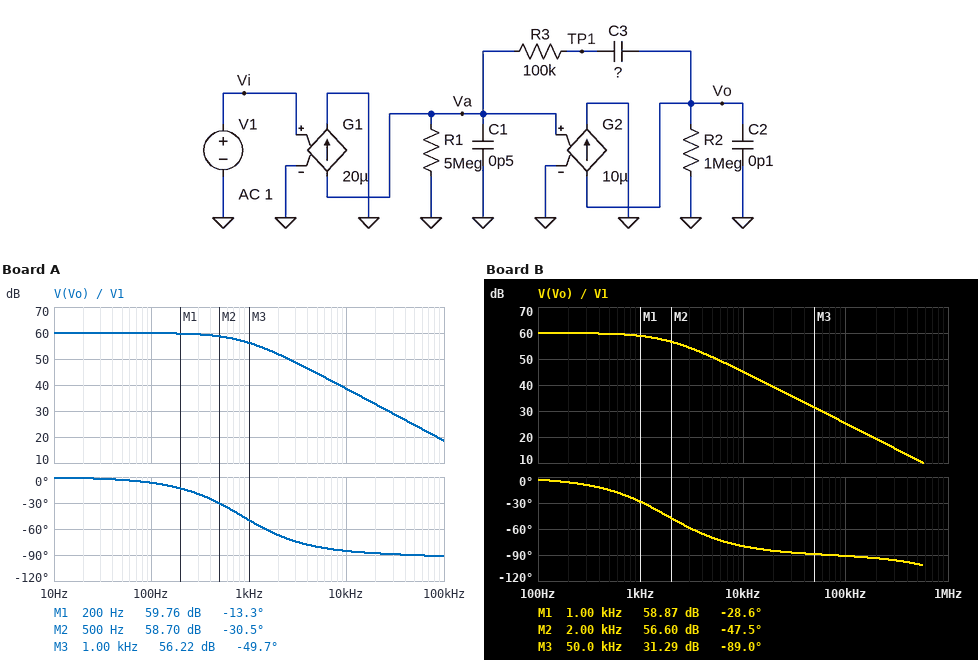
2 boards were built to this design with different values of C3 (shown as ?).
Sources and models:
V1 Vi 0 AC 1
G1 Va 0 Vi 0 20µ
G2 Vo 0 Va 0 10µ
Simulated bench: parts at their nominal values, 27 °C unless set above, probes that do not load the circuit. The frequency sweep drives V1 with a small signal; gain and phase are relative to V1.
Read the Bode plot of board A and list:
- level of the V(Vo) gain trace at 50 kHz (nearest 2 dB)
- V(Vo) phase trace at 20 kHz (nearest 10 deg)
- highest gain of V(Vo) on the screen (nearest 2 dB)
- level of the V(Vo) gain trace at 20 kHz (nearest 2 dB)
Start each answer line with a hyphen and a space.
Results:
- 24 dB
- -90 deg
- 60 dB
- 32 dB
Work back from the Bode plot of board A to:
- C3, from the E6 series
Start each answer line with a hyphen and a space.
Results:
- 3.3 pF
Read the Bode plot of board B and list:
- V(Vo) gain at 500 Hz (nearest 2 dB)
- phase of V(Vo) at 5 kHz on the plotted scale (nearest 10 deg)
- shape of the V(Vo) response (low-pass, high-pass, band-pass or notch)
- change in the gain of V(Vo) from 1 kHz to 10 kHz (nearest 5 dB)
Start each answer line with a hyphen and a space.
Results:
- 60 dB
- -70 deg
- low-pass
- -15 dB
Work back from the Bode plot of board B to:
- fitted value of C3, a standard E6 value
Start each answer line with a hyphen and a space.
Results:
- 1.5 pF
